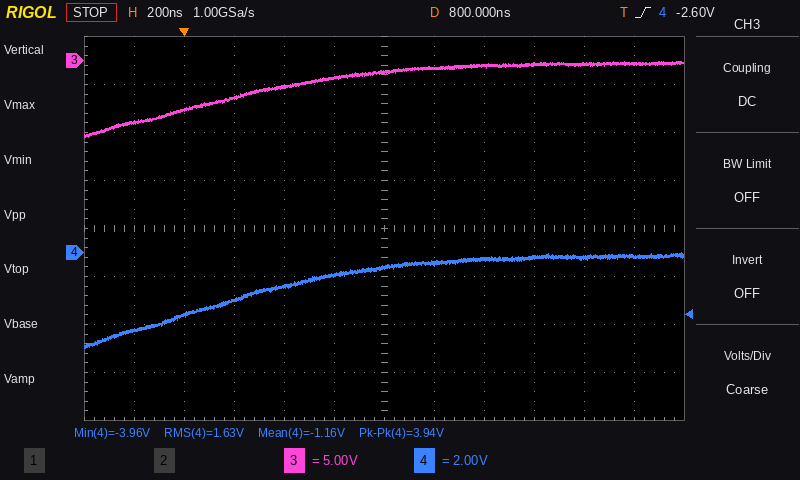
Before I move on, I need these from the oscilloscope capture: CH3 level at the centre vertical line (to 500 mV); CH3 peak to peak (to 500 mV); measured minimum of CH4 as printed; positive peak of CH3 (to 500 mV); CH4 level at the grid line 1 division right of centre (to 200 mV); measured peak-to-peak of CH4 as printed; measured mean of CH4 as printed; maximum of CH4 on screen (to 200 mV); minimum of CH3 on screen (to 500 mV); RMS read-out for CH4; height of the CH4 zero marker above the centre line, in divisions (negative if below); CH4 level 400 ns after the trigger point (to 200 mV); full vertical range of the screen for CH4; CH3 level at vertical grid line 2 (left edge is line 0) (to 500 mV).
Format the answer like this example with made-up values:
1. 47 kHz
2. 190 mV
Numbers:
1. -1.0 V
2. 8.0 V
3. -3.96 V
4. 0.0 V
5. -400 mV
6. 3.94 V
7. -1.16 V
8. 0.0 V
9. -8.0 V
10. 1.63 V
11. -0.5 div
12. -1.4 V
13. 16 V
14. -5.0 V
